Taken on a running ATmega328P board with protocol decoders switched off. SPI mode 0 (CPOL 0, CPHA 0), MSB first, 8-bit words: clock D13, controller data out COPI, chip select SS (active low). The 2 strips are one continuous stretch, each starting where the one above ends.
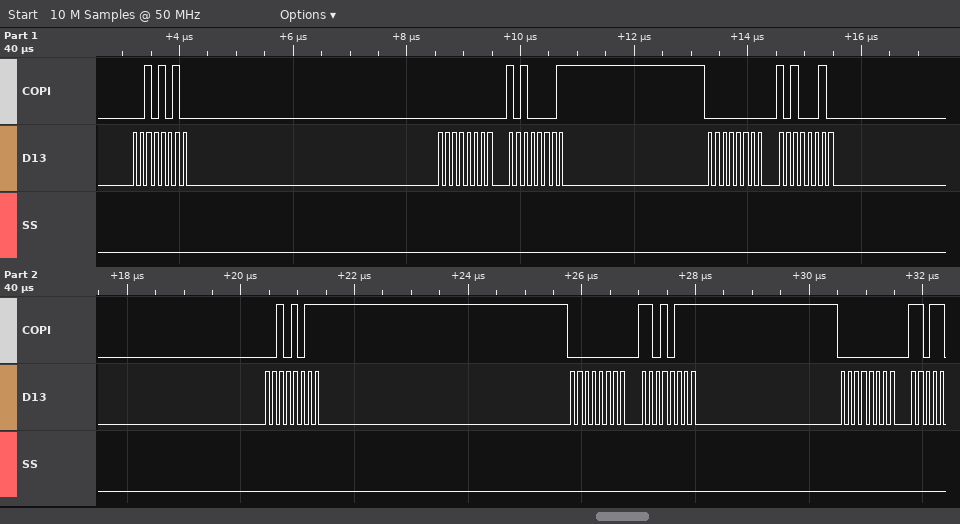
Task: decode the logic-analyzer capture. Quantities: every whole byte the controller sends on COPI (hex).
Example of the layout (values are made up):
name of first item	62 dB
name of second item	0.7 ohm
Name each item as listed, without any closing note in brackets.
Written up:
every whole byte the controller sends on COPI	2A 00 A1 00 A2 2B 00 D7 00
